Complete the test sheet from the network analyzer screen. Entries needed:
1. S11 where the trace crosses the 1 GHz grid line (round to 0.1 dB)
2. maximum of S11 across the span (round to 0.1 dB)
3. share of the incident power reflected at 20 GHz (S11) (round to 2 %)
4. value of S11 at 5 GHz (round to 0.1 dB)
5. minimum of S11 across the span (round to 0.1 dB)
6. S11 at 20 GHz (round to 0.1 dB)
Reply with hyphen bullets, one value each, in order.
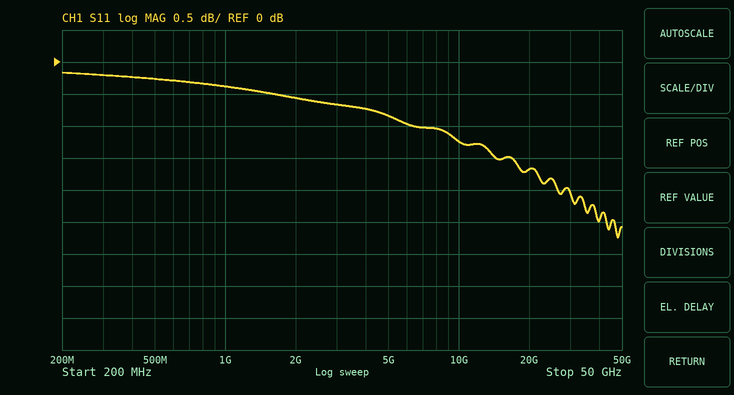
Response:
- -0.4 dB
- -0.2 dB
- 68 %
- -0.8 dB
- -2.7 dB
- -1.7 dB
